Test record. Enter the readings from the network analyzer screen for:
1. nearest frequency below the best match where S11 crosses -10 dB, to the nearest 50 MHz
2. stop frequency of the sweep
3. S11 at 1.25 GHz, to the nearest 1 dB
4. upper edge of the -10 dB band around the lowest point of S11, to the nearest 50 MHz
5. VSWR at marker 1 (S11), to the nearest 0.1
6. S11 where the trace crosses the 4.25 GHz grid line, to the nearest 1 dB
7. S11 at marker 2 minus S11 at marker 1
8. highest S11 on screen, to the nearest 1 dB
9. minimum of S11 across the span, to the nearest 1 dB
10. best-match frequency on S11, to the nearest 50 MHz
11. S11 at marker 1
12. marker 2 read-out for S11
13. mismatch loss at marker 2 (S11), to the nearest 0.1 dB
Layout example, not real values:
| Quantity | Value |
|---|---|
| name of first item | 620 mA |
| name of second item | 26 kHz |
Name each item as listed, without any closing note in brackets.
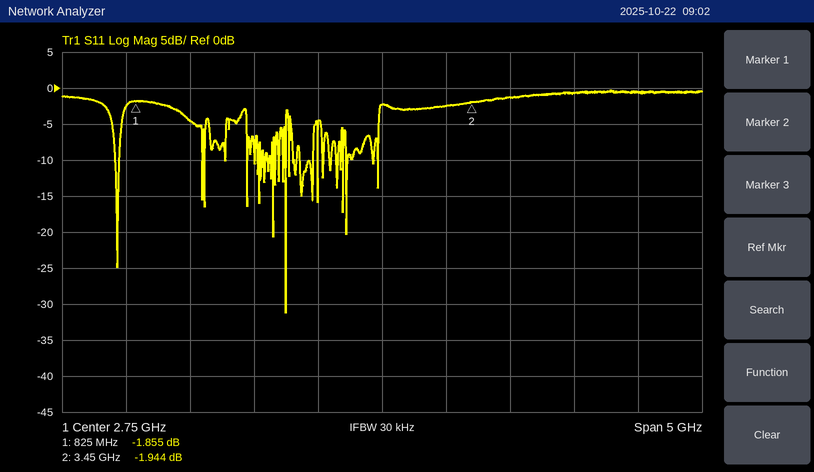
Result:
| Quantity | Value |
|---|---|
| nearest frequency below the best match where S11 crosses -10 dB, to the nearest 50 MHz | 2.00 GHz |
| stop frequency of the sweep | 5.25 GHz |
| S11 at 1.25 GHz, to the nearest 1 dB | -5 dB |
| upper edge of the -10 dB band around the lowest point of S11, to the nearest 50 MHz | 2.00 GHz |
| VSWR at marker 1 (S11), to the nearest 0.1 | 9.4 |
| S11 where the trace crosses the 4.25 GHz grid line, to the nearest 1 dB | -1 dB |
| S11 at marker 2 minus S11 at marker 1 | -0.089 dB |
| highest S11 on screen, to the nearest 1 dB | 0 dB |
| minimum of S11 across the span, to the nearest 1 dB | -31 dB |
| best-match frequency on S11, to the nearest 50 MHz | 2.00 GHz |
| S11 at marker 1 | -1.855 dB |
| marker 2 read-out for S11 | -1.944 dB |
| mismatch loss at marker 2 (S11), to the nearest 0.1 dB | 4.4 dB |
